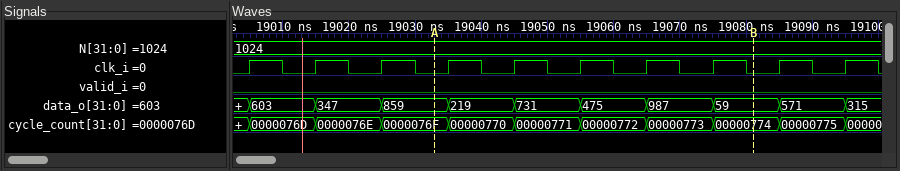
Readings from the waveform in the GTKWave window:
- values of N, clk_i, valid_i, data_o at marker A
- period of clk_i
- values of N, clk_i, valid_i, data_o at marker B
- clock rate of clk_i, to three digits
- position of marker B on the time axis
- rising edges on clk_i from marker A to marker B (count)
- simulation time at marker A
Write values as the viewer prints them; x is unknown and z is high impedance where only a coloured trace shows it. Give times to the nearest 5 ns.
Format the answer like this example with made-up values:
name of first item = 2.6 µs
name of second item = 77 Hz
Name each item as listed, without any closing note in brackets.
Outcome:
values of N, clk_i, valid_i, data_o at marker A = N=1024, clk_i=0, valid_i=0, data_o=859
period of clk_i = 10 ns
values of N, clk_i, valid_i, data_o at marker B = N=1024, clk_i=0, valid_i=0, data_o=59
clock rate of clk_i, to three digits = 100 MHz
position of marker B on the time axis = 19080 ns
rising edges on clk_i from marker A to marker B = 5
simulation time at marker A = 19035 ns
